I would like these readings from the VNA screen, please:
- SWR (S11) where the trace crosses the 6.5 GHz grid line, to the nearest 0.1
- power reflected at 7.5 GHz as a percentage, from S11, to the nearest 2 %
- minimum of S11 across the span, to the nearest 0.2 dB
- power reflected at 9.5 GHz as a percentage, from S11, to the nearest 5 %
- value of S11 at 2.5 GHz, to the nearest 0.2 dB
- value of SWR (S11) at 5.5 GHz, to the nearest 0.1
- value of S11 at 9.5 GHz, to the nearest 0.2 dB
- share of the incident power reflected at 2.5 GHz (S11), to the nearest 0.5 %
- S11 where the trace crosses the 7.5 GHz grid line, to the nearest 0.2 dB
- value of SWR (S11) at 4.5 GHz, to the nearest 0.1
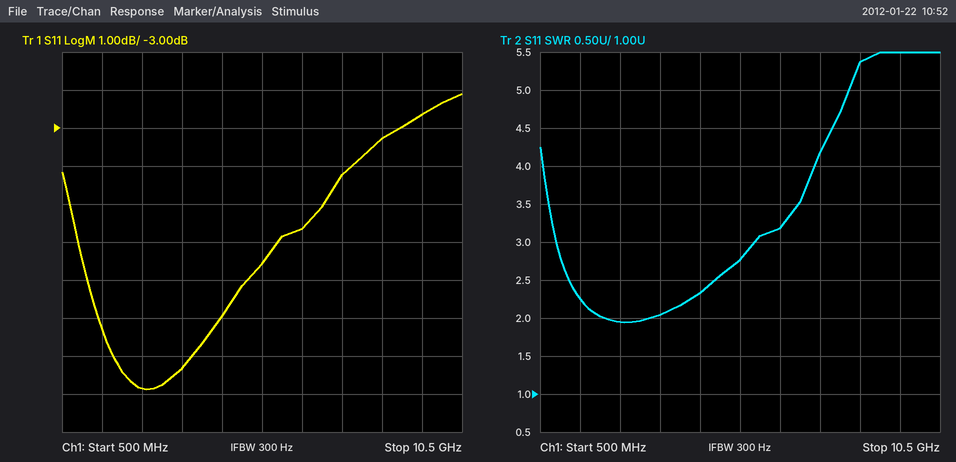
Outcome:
3.2
38 %
-9.8 dB
55 %
-9.8 dB
2.8
-2.6 dB
10.5 %
-4.2 dB
2.3
